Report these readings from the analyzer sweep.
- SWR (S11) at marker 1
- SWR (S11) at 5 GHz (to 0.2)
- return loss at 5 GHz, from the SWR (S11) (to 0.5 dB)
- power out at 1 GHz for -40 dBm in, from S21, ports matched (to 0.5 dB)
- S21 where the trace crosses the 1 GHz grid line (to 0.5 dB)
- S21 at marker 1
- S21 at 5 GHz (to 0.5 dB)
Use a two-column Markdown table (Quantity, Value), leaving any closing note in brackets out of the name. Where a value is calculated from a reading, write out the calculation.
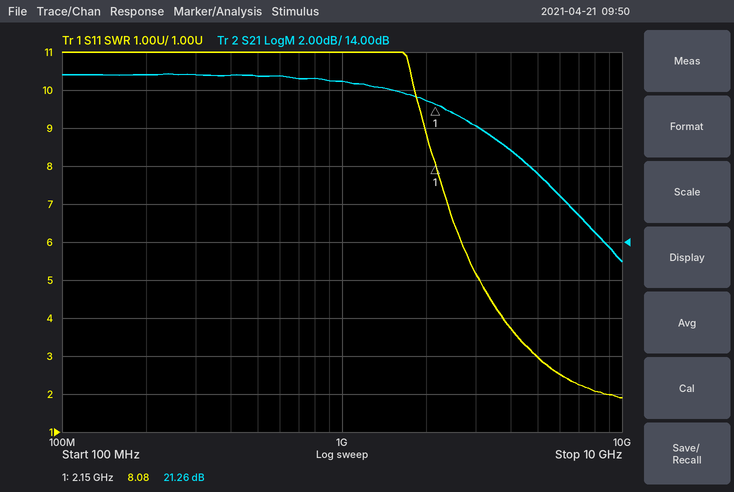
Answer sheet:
| Quantity | Value |
|---|---|
| SWR (S11) at marker 1 | 8.08 |
| SWR (S11) at 5 GHz | 3.0 |
| return loss at 5 GHz, from the SWR (S11) | −20 log10((3 − 1)/(3 + 1)) ≈ 6.0 dB |
| power out at 1 GHz for -40 dBm in, from S21, ports matched | -40 dBm + (22.5 dB) = -17.5 dBm |
| S21 where the trace crosses the 1 GHz grid line | 22.5 dB |
| S21 at marker 1 | 21.26 dB |
| S21 at 5 GHz | 17.5 dB |
